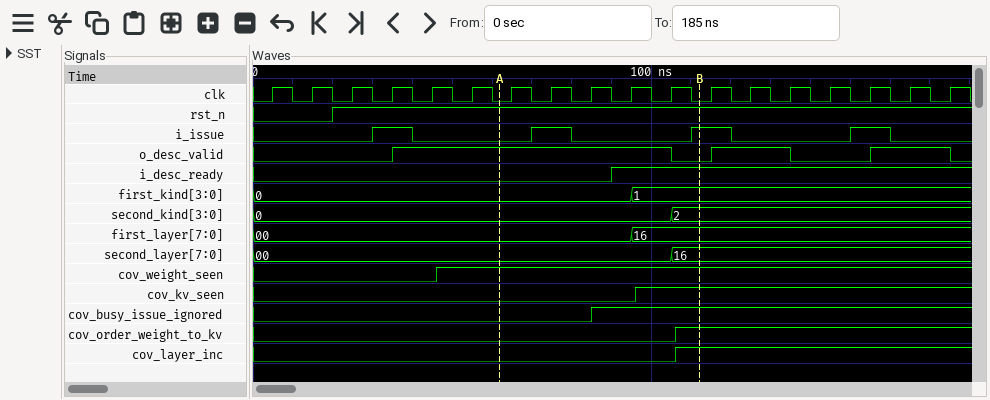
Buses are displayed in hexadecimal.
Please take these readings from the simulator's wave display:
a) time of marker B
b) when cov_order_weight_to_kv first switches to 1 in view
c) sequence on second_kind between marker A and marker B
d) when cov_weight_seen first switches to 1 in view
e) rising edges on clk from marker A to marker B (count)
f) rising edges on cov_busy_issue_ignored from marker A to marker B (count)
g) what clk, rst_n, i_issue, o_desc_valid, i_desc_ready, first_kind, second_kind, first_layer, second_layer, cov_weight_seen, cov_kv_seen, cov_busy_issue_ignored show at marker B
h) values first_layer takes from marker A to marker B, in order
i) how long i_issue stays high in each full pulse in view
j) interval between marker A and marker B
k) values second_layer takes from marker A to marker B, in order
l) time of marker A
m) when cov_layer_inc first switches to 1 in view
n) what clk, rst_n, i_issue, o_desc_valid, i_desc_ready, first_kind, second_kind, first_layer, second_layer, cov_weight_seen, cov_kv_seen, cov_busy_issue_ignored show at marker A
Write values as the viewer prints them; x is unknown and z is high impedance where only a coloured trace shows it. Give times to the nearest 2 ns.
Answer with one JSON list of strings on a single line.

["112 ns", "106 ns", "0, 2", "46 ns", "5", "1", "clk=0, rst_n=1, i_issue=1, o_desc_valid=0, i_desc_ready=1, first_kind=1, second_kind=2, first_layer=16, second_layer=16, cov_weight_seen=1, cov_kv_seen=1, cov_busy_issue_ignored=1", "00, 16", "10 ns, 10 ns, 10 ns, 10 ns", "50 ns", "00, 16", "62 ns", "106 ns", "clk=0, rst_n=1, i_issue=0, o_desc_valid=1, i_desc_ready=0, first_kind=0, second_kind=0, first_layer=00, second_layer=00, cov_weight_seen=1, cov_kv_seen=0, cov_busy_issue_ignored=0"]
